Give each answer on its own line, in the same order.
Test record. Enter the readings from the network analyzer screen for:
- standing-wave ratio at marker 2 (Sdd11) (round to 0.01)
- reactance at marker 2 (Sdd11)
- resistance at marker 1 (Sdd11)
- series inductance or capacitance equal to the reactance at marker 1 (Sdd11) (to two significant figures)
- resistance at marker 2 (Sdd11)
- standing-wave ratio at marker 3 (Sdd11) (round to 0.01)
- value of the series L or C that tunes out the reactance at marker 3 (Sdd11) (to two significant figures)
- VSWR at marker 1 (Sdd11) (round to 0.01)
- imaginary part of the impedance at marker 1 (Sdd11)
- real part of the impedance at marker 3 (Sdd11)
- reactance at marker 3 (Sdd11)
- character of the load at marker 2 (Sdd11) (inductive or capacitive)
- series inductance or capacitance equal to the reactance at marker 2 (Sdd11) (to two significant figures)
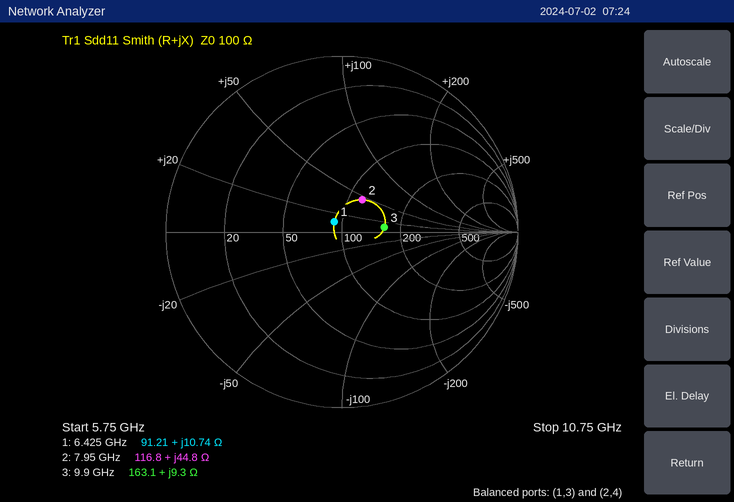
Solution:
1.55
+44.8 Ω
91.21 Ω
270 pH
116.8 Ω
1.64
1.7 pF
1.16
+10.74 Ω
163.1 Ω
+9.3 Ω
inductive
900 pH
